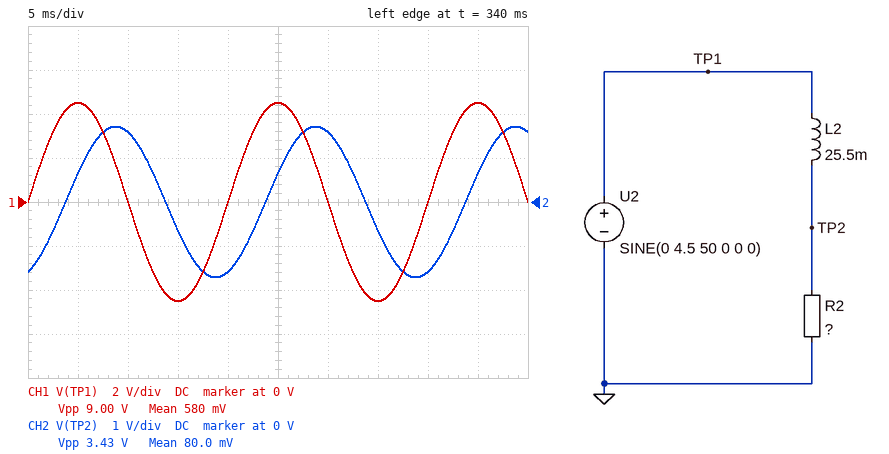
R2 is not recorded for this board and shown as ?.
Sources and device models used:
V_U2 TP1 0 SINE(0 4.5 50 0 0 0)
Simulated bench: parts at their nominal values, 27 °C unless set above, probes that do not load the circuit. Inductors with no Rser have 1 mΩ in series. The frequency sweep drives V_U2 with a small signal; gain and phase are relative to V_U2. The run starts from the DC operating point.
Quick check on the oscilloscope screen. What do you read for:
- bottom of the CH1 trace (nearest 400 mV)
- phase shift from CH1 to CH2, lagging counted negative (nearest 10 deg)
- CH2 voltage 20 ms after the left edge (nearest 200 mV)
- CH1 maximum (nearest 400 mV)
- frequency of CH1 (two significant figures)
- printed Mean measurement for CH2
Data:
-4.4 V
-70 deg
-1.6 V
4.4 V
50 Hz
80.0 mV
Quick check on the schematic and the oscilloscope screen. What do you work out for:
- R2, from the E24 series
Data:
3.3 Ω
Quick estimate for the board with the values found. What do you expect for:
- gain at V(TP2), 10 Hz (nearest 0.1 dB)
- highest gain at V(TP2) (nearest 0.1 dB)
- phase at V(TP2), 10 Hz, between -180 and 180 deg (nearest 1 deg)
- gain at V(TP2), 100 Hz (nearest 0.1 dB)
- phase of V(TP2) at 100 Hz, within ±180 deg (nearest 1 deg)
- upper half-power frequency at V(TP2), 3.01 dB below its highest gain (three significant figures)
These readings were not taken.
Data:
-0.9 dB
0 dB
-26 deg
-13.9 dB
-78 deg
20.6 Hz
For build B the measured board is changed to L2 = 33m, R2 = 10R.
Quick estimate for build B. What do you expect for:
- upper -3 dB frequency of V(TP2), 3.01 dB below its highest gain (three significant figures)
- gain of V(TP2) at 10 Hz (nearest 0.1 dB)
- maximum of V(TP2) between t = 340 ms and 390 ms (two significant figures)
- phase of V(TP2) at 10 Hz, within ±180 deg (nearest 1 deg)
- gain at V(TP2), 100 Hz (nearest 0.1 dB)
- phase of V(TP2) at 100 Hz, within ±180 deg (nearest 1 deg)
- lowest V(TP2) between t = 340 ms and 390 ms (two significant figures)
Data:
48.2 Hz
-0.2 dB
3.1 V
-12 deg
-7.2 dB
-64 deg
-3.1 V
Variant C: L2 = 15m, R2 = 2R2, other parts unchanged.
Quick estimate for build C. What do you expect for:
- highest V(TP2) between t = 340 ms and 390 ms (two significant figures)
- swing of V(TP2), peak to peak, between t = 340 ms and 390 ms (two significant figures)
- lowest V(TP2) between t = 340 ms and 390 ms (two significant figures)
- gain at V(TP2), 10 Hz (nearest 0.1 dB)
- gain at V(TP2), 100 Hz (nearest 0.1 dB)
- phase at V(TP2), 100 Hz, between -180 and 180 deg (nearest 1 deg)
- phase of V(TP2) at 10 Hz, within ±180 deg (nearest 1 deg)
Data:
1.9 V
3.8 V
-1.9 V
-0.7 dB
-12.9 dB
-77 deg
-23 deg
